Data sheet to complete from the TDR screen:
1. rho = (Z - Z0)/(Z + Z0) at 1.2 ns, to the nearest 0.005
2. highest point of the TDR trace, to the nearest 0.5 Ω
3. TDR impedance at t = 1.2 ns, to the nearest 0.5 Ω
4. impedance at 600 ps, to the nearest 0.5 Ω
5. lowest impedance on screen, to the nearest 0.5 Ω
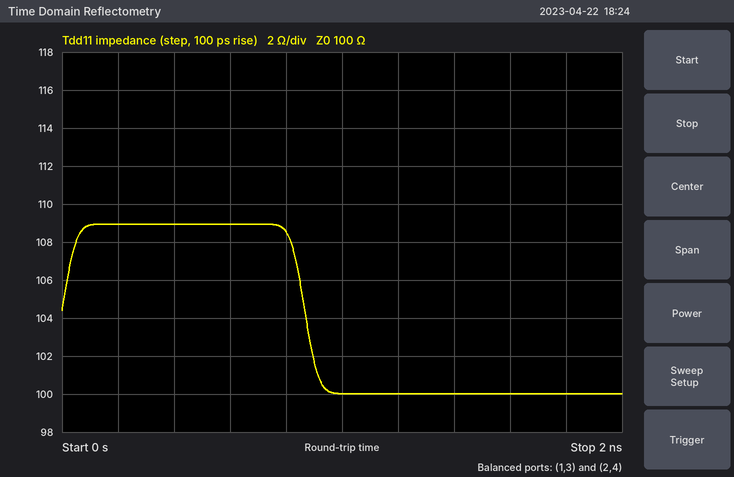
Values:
0.000
109.0 Ω
100.0 Ω
109.0 Ω
100.0 Ω
